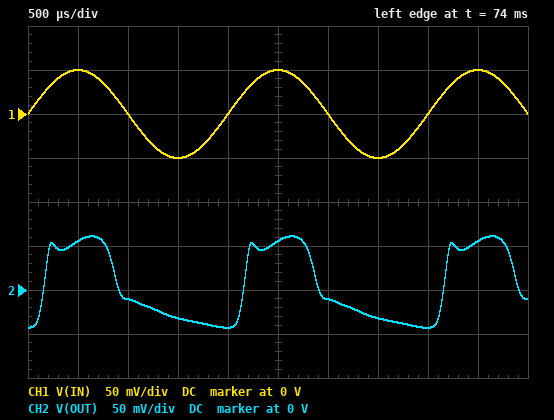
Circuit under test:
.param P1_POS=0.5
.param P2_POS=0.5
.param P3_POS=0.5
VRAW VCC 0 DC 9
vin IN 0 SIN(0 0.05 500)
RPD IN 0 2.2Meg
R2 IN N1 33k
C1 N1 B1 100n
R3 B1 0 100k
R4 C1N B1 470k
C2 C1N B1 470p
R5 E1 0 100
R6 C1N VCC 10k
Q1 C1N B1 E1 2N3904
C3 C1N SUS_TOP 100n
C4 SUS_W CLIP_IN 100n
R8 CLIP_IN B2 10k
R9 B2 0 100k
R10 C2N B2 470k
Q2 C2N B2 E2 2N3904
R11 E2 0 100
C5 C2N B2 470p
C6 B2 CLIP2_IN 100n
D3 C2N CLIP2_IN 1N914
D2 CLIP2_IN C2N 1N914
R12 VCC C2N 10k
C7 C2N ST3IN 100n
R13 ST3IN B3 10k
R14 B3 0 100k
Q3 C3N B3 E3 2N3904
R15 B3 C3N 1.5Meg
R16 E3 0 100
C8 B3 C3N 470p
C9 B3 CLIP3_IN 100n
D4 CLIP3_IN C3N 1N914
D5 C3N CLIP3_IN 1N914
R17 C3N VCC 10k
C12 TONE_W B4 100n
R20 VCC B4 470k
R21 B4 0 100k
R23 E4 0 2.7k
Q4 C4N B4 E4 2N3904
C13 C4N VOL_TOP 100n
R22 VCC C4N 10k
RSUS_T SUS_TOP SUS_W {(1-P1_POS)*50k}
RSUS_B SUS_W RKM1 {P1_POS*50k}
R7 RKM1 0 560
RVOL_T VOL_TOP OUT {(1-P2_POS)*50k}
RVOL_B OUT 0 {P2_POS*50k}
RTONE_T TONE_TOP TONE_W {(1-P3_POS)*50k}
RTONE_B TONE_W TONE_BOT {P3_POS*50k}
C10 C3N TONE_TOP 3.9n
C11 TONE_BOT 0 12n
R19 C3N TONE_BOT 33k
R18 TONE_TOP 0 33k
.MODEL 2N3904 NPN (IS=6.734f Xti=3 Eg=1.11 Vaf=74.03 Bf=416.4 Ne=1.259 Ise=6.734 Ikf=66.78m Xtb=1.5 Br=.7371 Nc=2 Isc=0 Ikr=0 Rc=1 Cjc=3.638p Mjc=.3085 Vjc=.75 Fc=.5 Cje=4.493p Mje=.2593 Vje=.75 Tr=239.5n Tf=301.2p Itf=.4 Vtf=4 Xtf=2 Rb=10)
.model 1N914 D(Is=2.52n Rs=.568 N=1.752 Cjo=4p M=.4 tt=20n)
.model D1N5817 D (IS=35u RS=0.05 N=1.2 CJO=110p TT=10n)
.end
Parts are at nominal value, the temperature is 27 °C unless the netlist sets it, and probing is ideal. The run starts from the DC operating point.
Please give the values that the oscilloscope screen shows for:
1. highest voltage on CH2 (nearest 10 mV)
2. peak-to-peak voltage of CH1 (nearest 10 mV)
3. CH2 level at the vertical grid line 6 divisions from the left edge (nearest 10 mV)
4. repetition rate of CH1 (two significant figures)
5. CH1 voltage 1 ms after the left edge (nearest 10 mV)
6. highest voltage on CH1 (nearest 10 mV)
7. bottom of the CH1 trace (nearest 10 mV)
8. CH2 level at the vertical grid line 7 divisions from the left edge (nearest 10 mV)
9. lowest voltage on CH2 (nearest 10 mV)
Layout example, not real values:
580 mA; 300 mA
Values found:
60 mV; 100 mV; -10 mV; 500 Hz; 0 V; 50 mV; -50 mV; -30 mV; -40 mV
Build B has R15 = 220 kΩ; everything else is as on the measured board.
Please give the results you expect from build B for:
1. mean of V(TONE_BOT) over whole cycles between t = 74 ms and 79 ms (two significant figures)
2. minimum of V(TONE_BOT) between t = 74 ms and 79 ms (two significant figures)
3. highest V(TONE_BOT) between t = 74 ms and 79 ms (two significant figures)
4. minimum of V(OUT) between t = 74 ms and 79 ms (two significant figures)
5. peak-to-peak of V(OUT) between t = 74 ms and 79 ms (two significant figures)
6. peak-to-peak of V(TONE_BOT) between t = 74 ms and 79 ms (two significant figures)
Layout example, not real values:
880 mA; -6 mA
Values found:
3.7 V; 3.5 V; 3.9 V; -140 mV; 270 mV; 450 mV
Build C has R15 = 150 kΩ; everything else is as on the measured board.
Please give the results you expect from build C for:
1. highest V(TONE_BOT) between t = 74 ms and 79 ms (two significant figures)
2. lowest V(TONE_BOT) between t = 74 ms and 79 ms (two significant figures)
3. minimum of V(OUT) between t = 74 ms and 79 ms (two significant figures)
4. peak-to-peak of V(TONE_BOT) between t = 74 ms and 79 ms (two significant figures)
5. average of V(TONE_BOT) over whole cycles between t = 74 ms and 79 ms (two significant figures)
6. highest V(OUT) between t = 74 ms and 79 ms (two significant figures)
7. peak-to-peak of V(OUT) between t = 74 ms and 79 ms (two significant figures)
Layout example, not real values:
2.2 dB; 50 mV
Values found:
3.3 V; 2.8 V; -140 mV; 440 mV; 3.1 V; 130 mV; 270 mV
